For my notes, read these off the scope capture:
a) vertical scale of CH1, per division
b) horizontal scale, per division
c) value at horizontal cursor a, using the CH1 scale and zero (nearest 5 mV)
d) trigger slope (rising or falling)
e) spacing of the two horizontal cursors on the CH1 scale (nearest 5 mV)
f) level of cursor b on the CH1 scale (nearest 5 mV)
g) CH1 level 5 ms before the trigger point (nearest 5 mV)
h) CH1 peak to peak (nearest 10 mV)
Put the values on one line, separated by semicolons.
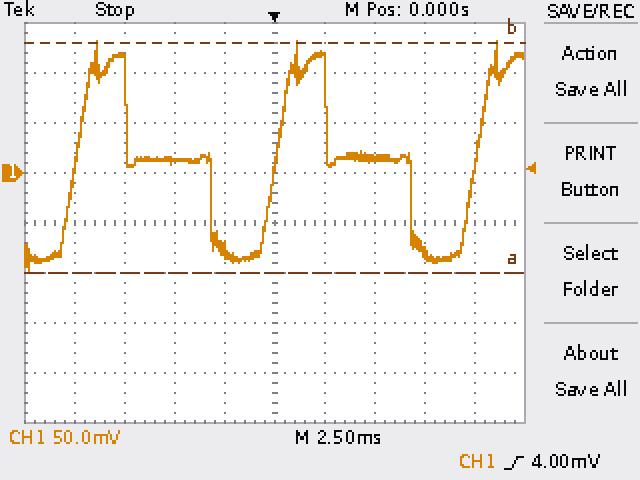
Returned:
50 mV; 2.5 ms; -100 mV; rising; 230 mV; 130 mV; 10 mV; 230 mV
